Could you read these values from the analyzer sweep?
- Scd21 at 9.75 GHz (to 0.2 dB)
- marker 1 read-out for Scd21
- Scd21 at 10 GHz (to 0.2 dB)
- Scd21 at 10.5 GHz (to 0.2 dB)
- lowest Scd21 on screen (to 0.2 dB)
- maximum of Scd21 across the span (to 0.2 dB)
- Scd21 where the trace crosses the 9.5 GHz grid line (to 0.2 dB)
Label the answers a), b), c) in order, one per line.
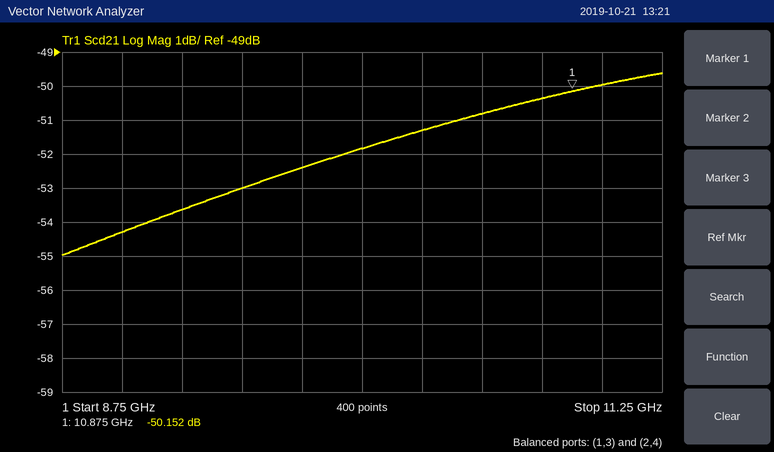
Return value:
a) -52.4 dB
b) -50.152 dB
c) -51.8 dB
d) -50.8 dB
e) -55.0 dB
f) -49.6 dB
g) -53.0 dB
